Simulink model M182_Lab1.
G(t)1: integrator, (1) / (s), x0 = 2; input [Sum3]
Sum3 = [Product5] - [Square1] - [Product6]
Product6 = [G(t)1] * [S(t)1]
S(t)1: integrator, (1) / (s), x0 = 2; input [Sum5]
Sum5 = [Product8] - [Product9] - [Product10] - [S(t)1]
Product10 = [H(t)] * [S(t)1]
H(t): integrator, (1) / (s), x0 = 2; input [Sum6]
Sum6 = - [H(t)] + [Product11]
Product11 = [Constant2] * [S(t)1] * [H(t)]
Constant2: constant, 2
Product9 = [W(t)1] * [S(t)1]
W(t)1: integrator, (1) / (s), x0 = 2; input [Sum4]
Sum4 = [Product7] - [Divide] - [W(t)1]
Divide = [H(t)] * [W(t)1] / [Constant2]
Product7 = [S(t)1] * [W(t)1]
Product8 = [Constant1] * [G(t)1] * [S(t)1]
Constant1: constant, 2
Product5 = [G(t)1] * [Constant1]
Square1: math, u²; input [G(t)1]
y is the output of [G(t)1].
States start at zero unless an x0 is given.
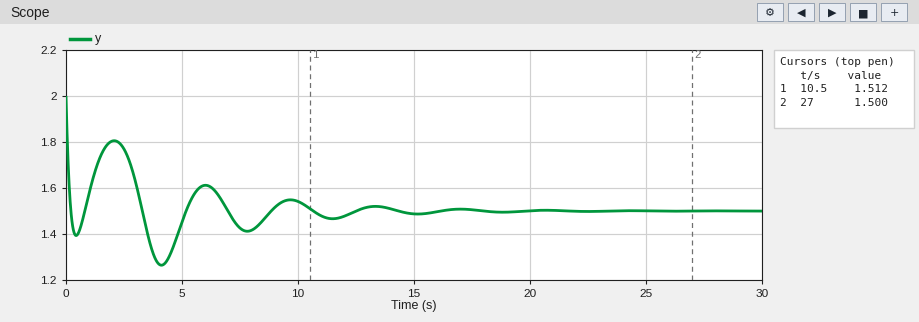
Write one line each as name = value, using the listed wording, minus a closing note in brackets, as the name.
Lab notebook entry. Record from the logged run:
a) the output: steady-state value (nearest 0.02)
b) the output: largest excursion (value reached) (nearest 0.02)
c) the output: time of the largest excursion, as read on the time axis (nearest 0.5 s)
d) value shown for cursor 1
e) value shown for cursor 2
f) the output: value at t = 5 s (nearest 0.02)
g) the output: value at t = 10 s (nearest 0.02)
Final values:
the output: steady-state value = 1.50
the output: largest excursion (value reached) = 1.26
the output: time of the largest excursion, as read on the time axis = 4.0 s
value shown for cursor 1 = 1.512
value shown for cursor 2 = 1.500
the output: value at t = 5 s = 1.46
the output: value at t = 10 s = 1.54
